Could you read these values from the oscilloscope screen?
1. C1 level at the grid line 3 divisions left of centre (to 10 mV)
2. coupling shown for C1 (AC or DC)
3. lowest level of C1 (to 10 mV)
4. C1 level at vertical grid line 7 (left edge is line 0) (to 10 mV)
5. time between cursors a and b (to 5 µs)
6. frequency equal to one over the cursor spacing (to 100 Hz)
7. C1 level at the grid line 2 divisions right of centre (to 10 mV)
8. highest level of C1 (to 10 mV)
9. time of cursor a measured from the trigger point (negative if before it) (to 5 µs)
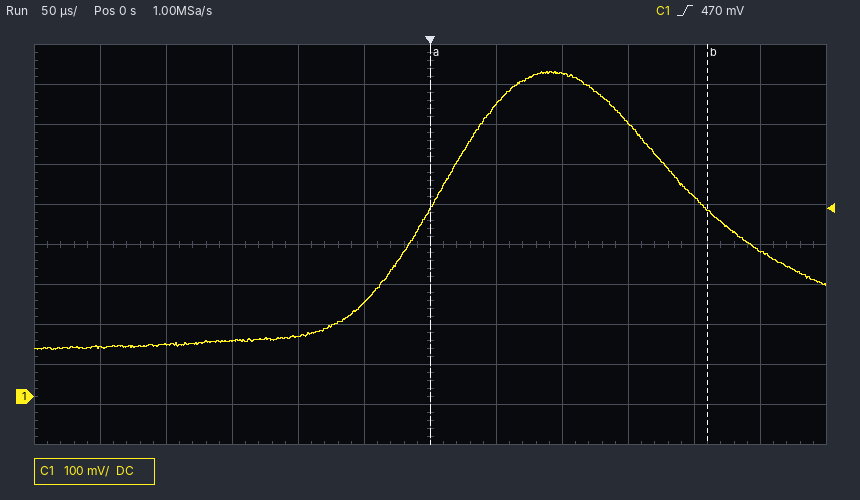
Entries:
140 mV
DC
120 mV
730 mV
210 µs
4.8 kHz
810 mV
810 mV
0 µs
